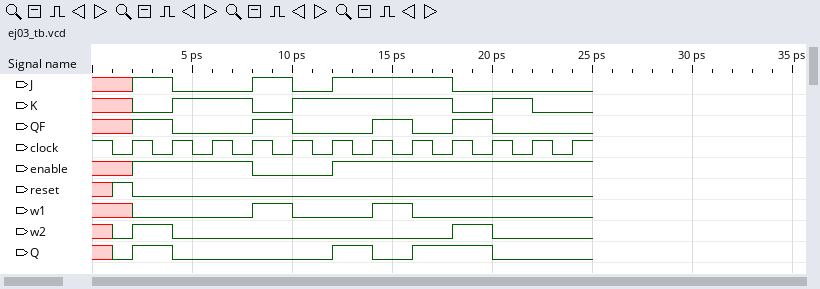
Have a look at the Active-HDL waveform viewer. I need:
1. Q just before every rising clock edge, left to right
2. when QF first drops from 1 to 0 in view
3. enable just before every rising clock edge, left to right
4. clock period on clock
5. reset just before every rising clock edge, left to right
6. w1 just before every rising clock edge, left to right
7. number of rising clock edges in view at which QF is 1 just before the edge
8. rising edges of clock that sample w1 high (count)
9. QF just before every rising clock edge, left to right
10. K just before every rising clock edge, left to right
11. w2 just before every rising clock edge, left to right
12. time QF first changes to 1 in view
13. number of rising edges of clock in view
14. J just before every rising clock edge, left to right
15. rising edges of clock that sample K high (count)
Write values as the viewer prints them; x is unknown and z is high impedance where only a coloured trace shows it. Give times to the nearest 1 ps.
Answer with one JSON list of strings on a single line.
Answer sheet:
["0 1 0 0 0 0 1 0 1 1 0 0", "4 ps", "x 1 1 1 0 0 1 1 1 1 1 1", "2 ps", "1 0 0 0 0 0 0 0 0 0 0 0", "x 0 0 0 1 0 0 1 0 0 0 0", "4", "2", "x 1 0 0 1 0 0 1 0 1 0 0", "x 0 1 1 0 1 1 1 1 0 1 0", "0 1 0 0 0 0 0 0 0 1 0 0", "2 ps", "12", "x 1 0 0 1 0 1 1 1 0 0 0", "7"]
